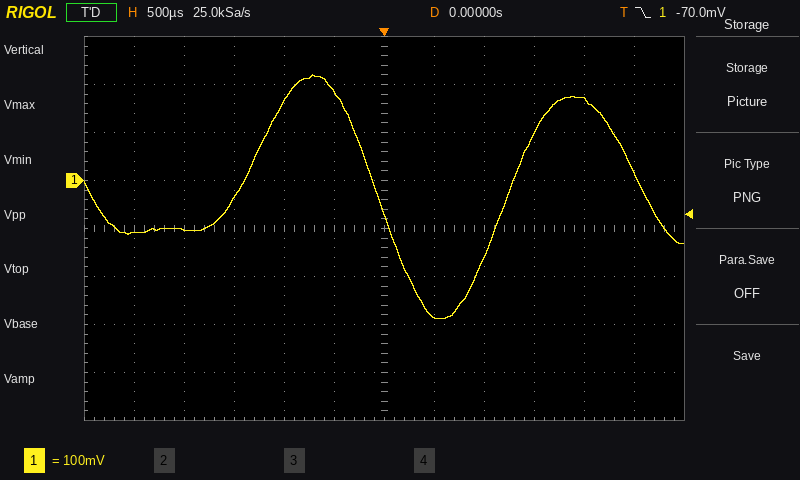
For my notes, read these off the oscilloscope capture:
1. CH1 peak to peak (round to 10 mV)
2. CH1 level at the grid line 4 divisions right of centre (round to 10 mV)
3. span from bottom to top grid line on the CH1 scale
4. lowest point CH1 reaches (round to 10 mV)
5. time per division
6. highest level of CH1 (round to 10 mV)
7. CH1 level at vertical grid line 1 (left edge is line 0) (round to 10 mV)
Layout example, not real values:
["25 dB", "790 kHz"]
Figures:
["510 mV", "170 mV", "800 mV", "-290 mV", "500 µs", "220 mV", "-110 mV"]
